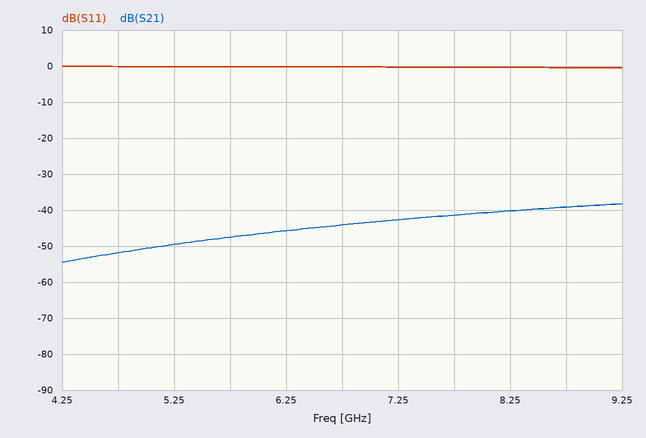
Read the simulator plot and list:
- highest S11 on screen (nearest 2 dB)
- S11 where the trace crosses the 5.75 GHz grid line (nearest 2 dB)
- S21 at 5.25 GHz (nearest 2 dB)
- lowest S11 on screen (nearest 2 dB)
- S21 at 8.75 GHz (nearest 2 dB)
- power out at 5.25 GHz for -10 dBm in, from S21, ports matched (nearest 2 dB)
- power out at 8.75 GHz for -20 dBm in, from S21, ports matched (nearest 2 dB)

0 dB
0 dB
-50 dB
0 dB
-40 dB
-60 dBm
-60 dBm
